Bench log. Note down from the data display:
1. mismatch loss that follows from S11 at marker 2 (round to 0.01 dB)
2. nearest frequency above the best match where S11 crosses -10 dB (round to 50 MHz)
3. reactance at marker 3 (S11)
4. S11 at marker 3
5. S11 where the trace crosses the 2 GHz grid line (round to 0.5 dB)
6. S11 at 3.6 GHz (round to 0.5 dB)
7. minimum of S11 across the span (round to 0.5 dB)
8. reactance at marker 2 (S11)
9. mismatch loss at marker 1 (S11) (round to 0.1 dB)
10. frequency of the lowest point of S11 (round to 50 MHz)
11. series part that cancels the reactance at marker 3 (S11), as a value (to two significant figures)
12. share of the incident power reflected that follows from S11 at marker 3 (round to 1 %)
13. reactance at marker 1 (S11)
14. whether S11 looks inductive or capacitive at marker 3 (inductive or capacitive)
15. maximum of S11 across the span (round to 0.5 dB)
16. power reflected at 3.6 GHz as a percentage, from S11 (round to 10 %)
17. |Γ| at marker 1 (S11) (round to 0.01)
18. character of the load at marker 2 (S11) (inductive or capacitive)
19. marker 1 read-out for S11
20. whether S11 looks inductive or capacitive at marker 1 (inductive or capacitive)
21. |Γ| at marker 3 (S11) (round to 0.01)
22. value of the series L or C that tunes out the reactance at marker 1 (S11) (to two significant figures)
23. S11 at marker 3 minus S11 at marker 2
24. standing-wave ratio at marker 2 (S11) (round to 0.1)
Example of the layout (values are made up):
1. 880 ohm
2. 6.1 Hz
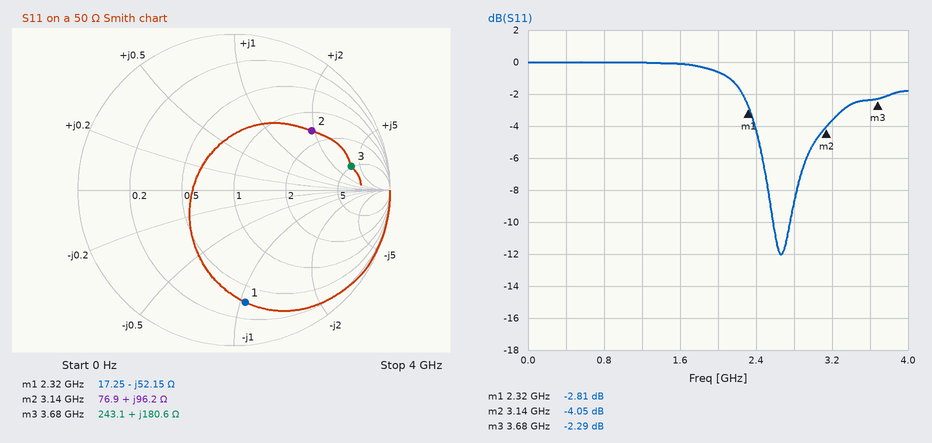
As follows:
1. 2.17 dB
2. 2.75 GHz
3. +180.6 Ω
4. -2.29 dB
5. -0.5 dB
6. -2.5 dB
7. -12.0 dB
8. +96.2 Ω
9. 3.2 dB
10. 2.65 GHz
11. 240 fF
12. 59 %
13. -52.15 Ω
14. inductive
15. 0.0 dB
16. 60 %
17. 0.72
18. inductive
19. -2.81 dB
20. capacitive
21. 0.77
22. 3.6 nH
23. 1.76 dB
24. 4.4
